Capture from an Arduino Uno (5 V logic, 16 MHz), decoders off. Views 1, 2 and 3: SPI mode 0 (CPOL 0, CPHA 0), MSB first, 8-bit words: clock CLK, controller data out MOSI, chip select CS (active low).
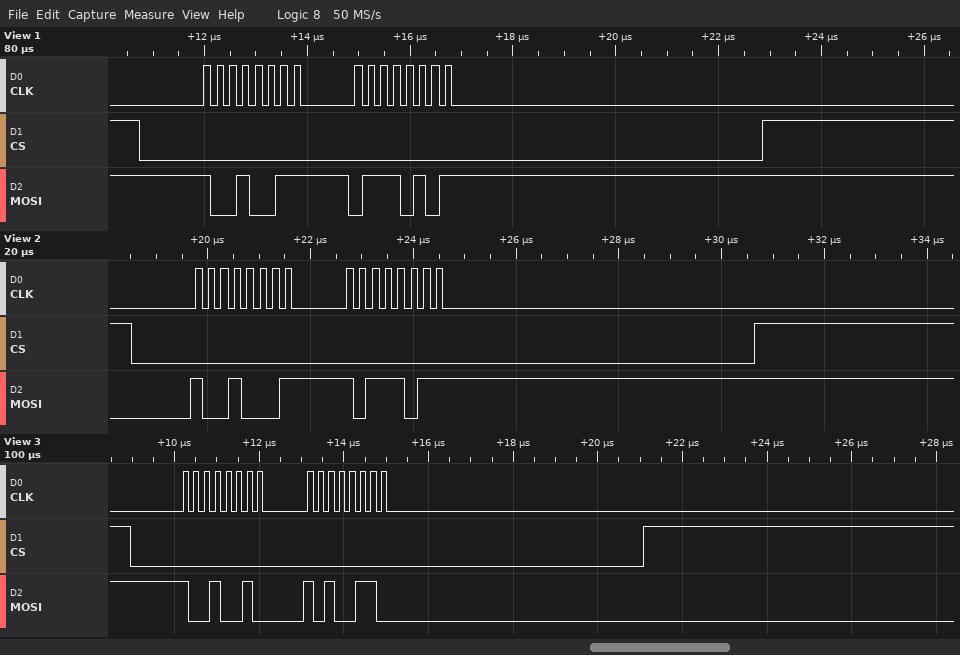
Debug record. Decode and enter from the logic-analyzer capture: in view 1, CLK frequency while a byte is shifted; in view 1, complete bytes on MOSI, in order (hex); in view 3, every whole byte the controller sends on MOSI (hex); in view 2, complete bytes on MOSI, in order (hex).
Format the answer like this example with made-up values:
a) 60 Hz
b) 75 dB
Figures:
a) 4 MHz
b) 93 75
c) 92 A6
d) 91 BB
